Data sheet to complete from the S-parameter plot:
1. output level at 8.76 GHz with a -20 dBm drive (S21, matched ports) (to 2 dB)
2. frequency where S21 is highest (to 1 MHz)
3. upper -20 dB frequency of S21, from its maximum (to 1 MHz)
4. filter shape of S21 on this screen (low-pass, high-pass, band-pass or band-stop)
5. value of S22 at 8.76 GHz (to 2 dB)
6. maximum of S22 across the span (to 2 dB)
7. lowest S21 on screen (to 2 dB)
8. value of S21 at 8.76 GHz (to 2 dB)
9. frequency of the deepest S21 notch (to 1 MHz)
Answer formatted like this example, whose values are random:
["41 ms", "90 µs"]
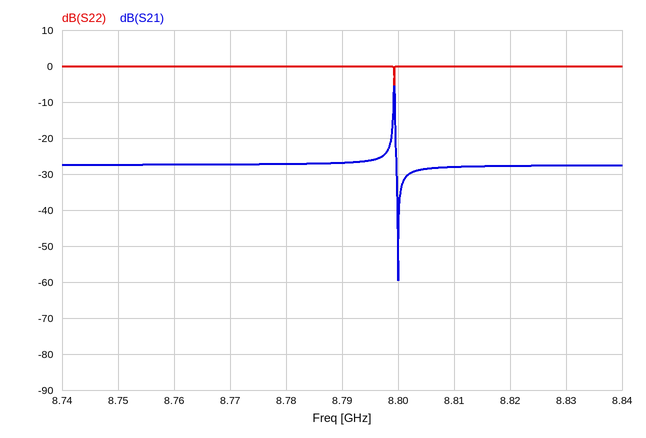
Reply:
["-48 dBm", "8.799 GHz", "8.800 GHz", "band-pass", "0 dB", "0 dB", "-60 dB", "-28 dB", "8.800 GHz"]
